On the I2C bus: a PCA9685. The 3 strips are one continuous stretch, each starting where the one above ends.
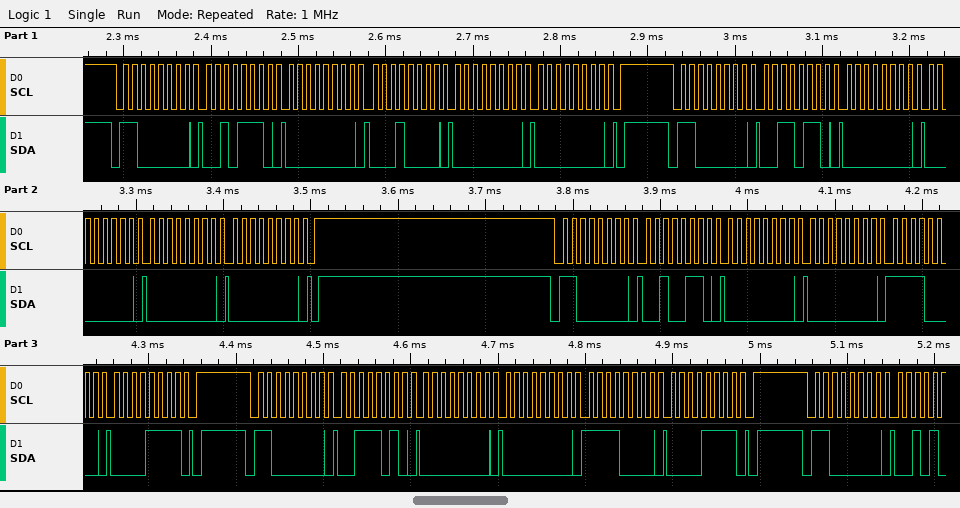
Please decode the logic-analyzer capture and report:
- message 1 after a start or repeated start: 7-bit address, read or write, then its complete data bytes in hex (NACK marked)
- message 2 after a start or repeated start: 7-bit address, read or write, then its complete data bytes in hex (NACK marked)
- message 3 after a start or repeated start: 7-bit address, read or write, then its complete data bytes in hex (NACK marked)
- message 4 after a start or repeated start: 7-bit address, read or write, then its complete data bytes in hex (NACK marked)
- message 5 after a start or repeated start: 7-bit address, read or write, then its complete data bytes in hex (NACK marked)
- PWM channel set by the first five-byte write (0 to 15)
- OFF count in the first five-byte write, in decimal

0x60 write: 2E 00 10 00 00
0x60 write: 36 00 00 00 00
0x60 write: 26 00 00 F0 0F
0x60 write: 3A 00 00 F0 0F
0x60 write
10
0
